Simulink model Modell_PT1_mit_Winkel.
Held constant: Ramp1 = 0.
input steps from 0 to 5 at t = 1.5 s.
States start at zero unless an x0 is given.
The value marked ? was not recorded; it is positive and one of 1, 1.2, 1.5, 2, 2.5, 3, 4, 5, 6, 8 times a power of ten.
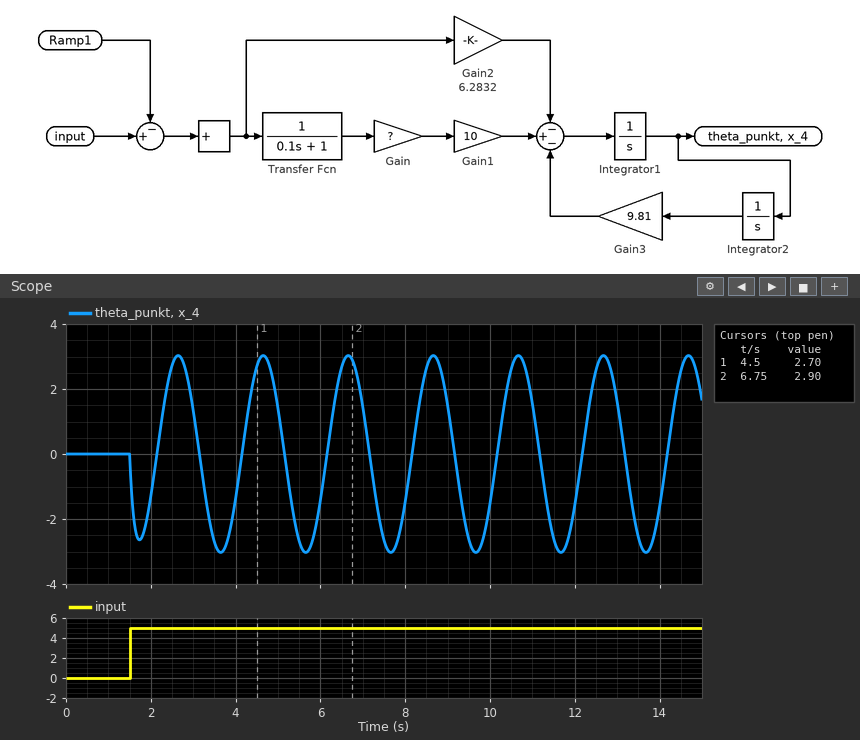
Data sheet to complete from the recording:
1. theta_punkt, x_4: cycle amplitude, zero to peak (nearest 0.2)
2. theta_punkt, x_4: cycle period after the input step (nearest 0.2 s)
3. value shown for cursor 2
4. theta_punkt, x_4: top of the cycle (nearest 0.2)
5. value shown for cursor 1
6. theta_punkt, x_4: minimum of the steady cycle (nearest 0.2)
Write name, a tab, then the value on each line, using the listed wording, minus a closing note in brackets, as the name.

theta_punkt, x_4: cycle amplitude, zero to peak	3.0
theta_punkt, x_4: cycle period after the input step	2.0 s
value shown for cursor 2	2.90
theta_punkt, x_4: top of the cycle	3.0
value shown for cursor 1	2.70
theta_punkt, x_4: minimum of the steady cycle	-3.0
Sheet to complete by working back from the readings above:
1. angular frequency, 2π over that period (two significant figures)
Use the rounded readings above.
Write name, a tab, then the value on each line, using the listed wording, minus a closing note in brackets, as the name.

angular frequency, 2π over that period	3.1 rad/s
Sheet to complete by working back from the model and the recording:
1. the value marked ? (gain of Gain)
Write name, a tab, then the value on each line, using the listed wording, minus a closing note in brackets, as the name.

the value marked ?	0.6
